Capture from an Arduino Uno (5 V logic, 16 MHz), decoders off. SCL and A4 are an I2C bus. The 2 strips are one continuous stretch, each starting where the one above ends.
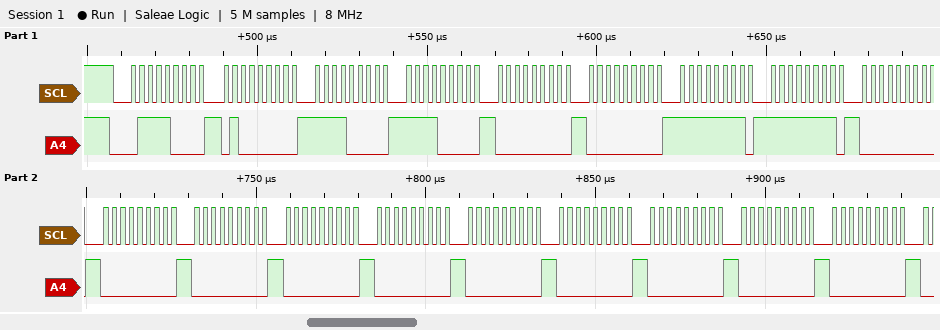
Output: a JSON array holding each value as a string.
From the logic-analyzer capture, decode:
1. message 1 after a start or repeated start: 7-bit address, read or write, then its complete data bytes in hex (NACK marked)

["0x3C write: 40 F0 F0 00 00 FF FF 00 00 00 00 00 00 00 00 00 00"]
